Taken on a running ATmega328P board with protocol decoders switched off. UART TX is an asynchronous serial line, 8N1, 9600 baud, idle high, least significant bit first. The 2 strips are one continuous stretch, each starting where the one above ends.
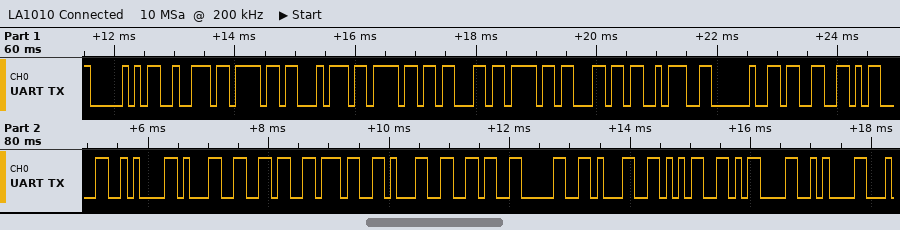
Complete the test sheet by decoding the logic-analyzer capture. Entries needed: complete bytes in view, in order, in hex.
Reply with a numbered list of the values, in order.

1. 50 72 6F 74 6F 63 6F 6C 3A 20 33 0D 0A 31 36 37 31 36 30 31 35 0D 0A
